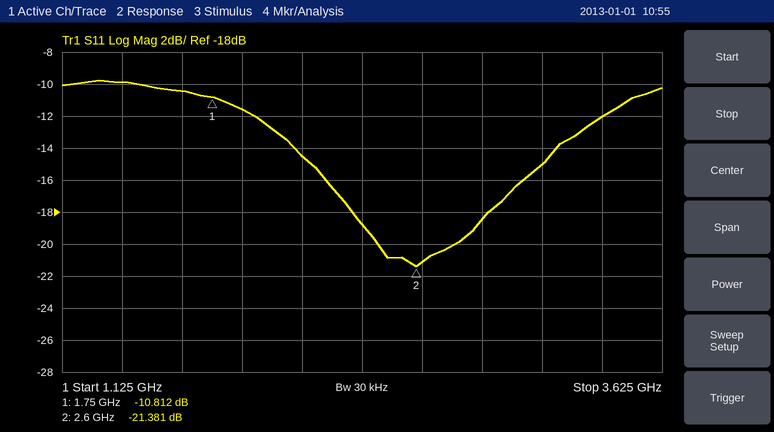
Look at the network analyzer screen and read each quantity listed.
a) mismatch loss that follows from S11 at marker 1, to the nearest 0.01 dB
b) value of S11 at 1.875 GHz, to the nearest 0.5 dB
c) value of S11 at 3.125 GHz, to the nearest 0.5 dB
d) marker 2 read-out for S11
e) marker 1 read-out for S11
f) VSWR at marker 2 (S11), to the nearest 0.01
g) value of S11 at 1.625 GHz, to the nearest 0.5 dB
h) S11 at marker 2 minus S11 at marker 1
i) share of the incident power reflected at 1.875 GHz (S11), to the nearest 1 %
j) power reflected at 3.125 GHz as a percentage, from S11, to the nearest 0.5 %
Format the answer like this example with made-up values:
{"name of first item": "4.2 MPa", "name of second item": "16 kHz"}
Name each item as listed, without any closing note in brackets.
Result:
{"mismatch loss that follows from S11 at marker 1, to the nearest 0.01 dB": "0.38 dB", "value of S11 at 1.875 GHz, to the nearest 0.5 dB": "-11.5 dB", "value of S11 at 3.125 GHz, to the nearest 0.5 dB": "-15.0 dB", "marker 2 read-out for S11": "-21.381 dB", "marker 1 read-out for S11": "-10.812 dB", "VSWR at marker 2 (S11), to the nearest 0.01": "1.19", "value of S11 at 1.625 GHz, to the nearest 0.5 dB": "-10.5 dB", "S11 at marker 2 minus S11 at marker 1": "-10.569 dB", "share of the incident power reflected at 1.875 GHz (S11), to the nearest 1 %": "7 %", "power reflected at 3.125 GHz as a percentage, from S11, to the nearest 0.5 %": "3.0 %"}
